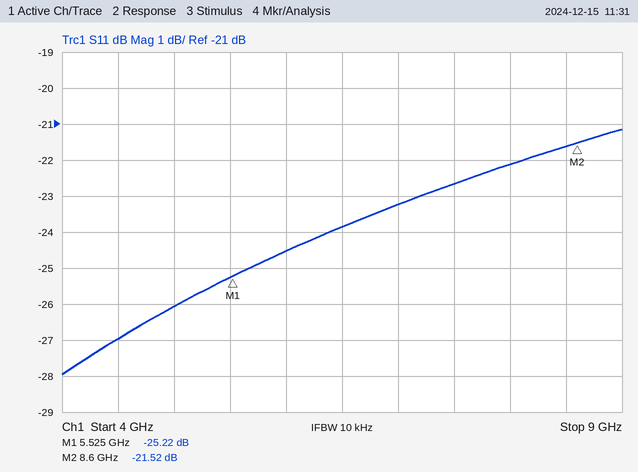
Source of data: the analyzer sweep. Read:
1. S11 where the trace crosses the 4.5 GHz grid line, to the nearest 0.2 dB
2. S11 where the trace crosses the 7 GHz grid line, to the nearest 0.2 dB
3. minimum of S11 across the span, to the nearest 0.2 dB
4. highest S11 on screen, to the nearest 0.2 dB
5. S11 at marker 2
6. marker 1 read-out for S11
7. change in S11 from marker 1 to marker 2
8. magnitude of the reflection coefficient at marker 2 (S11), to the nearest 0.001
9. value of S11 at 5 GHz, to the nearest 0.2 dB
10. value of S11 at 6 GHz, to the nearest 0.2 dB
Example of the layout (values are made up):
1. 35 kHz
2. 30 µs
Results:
1. -27.0 dB
2. -23.2 dB
3. -28.0 dB
4. -21.2 dB
5. -21.52 dB
6. -25.22 dB
7. 3.70 dB
8. 0.084
9. -26.0 dB
10. -24.6 dB
